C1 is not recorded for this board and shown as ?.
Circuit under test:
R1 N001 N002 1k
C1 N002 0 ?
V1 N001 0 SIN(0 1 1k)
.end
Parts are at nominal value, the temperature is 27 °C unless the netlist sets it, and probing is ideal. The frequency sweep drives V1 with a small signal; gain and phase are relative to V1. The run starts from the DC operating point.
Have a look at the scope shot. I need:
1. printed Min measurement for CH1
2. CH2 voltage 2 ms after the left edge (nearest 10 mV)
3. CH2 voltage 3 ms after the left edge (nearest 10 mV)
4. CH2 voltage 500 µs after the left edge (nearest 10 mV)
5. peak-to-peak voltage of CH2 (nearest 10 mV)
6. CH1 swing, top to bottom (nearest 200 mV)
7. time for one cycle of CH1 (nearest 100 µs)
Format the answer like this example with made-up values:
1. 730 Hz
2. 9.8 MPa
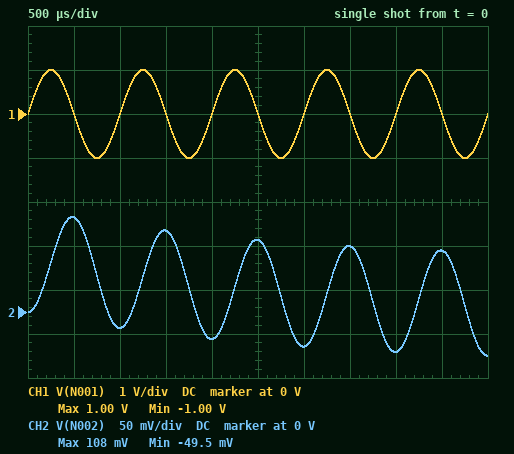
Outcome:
1. -1.00 V
2. -30 mV
3. -40 mV
4. 110 mV
5. 160 mV
6. 2.0 V
7. 1.0 ms
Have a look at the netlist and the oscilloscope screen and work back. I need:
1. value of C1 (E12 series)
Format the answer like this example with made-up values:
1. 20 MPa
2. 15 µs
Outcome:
1. 2.7 µF
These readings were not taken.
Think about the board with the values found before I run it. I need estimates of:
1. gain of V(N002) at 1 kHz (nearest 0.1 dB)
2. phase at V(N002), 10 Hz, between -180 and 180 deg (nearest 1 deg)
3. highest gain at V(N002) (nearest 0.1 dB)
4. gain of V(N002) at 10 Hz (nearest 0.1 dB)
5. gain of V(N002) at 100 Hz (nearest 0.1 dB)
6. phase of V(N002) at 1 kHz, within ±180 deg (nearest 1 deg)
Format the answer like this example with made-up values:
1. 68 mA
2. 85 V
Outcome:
1. -24.6 dB
2. -10 deg
3. 0 dB
4. -0.1 dB
5. -5.9 dB
6. -87 deg
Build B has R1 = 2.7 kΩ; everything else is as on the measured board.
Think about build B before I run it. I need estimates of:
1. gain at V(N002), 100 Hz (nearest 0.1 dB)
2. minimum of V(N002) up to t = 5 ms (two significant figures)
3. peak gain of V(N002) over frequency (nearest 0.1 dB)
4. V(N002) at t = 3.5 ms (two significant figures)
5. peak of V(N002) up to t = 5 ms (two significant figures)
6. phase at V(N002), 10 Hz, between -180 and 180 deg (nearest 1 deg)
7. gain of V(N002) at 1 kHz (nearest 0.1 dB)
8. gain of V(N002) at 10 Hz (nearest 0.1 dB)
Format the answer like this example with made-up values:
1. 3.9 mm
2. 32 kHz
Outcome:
1. -13.4 dB
2. -11 mV
3. 0 dB
4. 35 mV
5. 42 mV
6. -25 deg
7. -33.2 dB
8. -0.8 dB
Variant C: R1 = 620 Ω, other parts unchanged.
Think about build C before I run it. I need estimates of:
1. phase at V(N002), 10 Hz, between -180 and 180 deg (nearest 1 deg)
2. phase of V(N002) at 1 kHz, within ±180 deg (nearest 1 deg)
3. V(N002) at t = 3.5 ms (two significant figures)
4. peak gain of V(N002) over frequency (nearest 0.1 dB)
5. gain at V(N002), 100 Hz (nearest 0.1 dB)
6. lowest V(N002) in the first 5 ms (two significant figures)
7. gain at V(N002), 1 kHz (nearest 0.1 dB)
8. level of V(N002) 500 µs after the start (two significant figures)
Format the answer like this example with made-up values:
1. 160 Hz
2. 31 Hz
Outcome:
1. -6 deg
2. -85 deg
3. 110 mV
4. 0 dB
5. -3.2 dB
6. -90 mV
7. -20.5 dB
8. 160 mV
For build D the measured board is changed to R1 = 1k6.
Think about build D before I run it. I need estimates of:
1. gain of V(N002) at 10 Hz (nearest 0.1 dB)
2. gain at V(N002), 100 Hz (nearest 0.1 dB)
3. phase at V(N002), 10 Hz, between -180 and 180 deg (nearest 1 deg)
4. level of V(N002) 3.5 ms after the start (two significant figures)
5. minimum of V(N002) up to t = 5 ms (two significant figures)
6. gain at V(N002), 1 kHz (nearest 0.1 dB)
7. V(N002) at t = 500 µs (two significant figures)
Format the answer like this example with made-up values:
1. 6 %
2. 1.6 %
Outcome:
1. -0.3 dB
2. -9.2 dB
3. -15 deg
4. 53 mV
5. -25 mV
6. -28.7 dB
7. 70 mV
